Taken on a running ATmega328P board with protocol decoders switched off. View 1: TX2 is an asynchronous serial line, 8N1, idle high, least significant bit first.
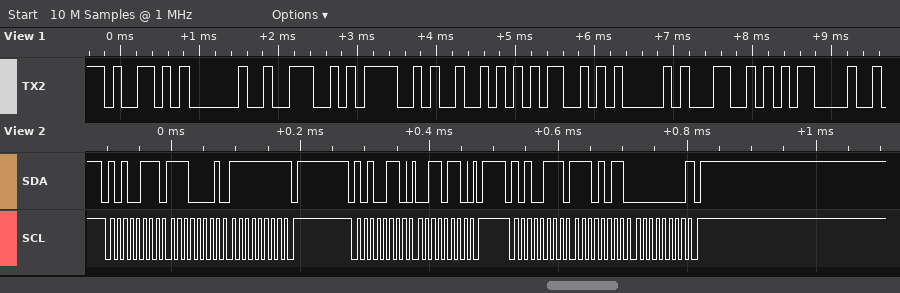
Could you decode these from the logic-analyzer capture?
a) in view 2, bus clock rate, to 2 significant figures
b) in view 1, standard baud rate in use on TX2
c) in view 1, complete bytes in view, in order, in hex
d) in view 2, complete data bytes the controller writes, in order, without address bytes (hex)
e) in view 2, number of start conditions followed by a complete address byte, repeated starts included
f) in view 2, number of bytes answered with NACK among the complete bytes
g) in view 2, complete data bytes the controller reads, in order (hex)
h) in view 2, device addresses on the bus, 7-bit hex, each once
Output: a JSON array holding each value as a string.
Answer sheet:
["100 kHz", "9600 baud", "59 20 4E 4F 52 4D 41 4C 0D", "36", "3", "2", "E1 FF EB 00", "0x53"]
